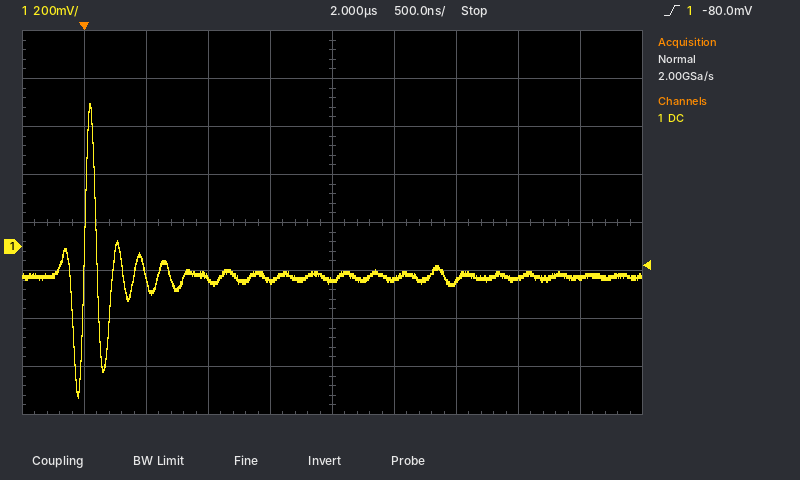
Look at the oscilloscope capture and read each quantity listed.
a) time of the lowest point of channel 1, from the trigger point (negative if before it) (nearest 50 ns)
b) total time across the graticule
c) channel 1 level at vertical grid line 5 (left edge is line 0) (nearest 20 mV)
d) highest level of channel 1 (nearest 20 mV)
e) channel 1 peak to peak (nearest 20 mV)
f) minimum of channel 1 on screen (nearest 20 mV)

-50 ns
5 µs
-140 mV
600 mV
1.22 V
-620 mV
